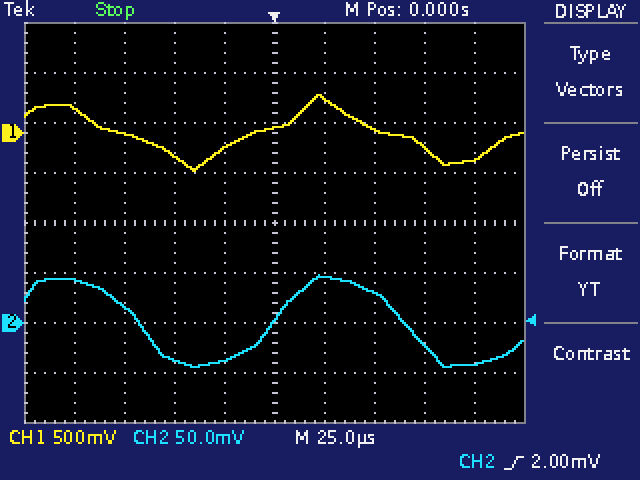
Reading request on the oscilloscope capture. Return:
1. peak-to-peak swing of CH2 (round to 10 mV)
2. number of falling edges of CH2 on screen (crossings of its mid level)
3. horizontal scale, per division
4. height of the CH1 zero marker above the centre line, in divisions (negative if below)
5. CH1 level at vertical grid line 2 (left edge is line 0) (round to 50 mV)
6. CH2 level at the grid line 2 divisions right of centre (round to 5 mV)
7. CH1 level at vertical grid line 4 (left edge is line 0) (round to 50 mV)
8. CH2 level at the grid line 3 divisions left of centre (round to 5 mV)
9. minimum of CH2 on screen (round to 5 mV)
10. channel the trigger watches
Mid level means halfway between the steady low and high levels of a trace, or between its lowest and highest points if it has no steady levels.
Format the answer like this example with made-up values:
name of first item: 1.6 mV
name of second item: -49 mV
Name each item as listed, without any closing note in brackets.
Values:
peak-to-peak swing of CH2: 90 mV
number of falling edges of CH2 on screen: 2
horizontal scale, per division: 25 µs
height of the CH1 zero marker above the centre line, in divisions: +1.8 div
CH1 level at vertical grid line 2 (left edge is line 0): 0 mV
CH2 level at the grid line 2 divisions right of centre: 30 mV
CH1 level at vertical grid line 4 (left edge is line 0): -150 mV
CH2 level at the grid line 3 divisions left of centre: 15 mV
minimum of CH2 on screen: -45 mV
channel the trigger watches: CH2
